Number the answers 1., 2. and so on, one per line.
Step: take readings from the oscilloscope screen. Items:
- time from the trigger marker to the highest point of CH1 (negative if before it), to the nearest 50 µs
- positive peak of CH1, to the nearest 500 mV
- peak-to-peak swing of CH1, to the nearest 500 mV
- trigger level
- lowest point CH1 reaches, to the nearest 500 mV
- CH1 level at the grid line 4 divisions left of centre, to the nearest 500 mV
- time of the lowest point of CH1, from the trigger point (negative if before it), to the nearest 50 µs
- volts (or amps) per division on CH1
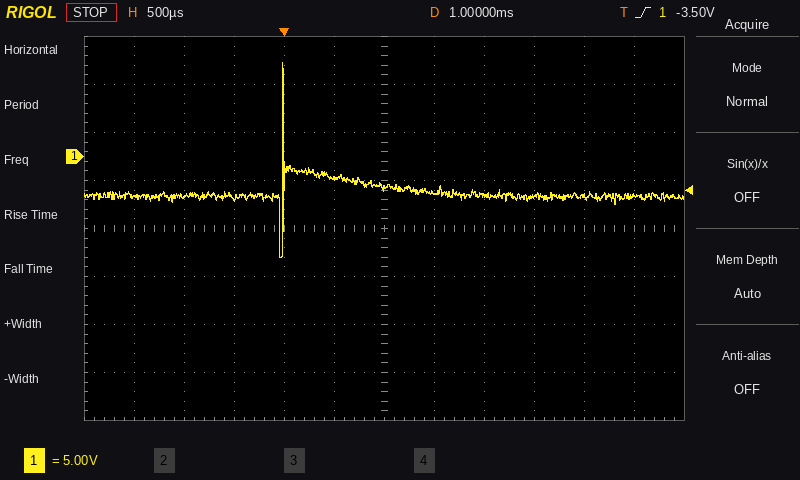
1. 0 µs
2. 10.0 V
3. 20.5 V
4. -3.50 V
5. -10.5 V
6. -4.0 V
7. -50 µs
8. 5 V
